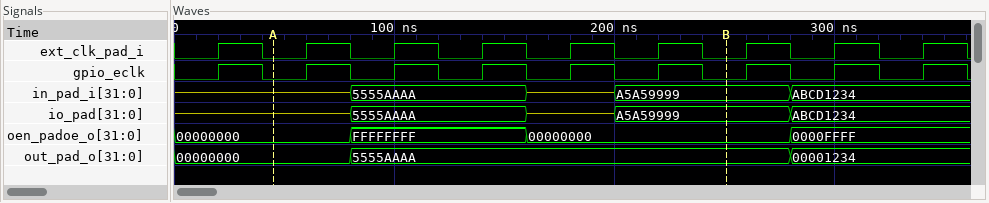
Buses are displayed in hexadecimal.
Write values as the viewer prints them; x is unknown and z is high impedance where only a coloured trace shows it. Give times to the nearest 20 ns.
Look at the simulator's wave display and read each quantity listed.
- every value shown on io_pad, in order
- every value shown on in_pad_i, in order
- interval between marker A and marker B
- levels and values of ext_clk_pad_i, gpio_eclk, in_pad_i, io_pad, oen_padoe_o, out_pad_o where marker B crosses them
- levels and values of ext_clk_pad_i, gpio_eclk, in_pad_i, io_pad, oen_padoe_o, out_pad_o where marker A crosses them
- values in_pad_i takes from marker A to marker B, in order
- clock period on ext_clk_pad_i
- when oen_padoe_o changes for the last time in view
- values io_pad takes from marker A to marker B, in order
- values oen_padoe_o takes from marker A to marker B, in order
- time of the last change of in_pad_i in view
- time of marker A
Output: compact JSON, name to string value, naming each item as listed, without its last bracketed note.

{"every value shown on io_pad, in order": "z, 5555AAAA, z, A5A59999, ABCD1234", "every value shown on in_pad_i, in order": "z, 5555AAAA, z, A5A59999, ABCD1234", "interval between marker A and marker B": "200 ns", "levels and values of ext_clk_pad_i, gpio_eclk, in_pad_i, io_pad, oen_padoe_o, out_pad_o where marker B crosses them": "ext_clk_pad_i=0, gpio_eclk=0, in_pad_i=A5A59999, io_pad=A5A59999, oen_padoe_o=00000000, out_pad_o=5555AAAA", "levels and values of ext_clk_pad_i, gpio_eclk, in_pad_i, io_pad, oen_padoe_o, out_pad_o where marker A crosses them": "ext_clk_pad_i=0, gpio_eclk=0, in_pad_i=z, io_pad=z, oen_padoe_o=00000000, out_pad_o=00000000", "values in_pad_i takes from marker A to marker B, in order": "z, 5555AAAA, z, A5A59999", "clock period on ext_clk_pad_i": "40 ns", "when oen_padoe_o changes for the last time in view": "280 ns", "values io_pad takes from marker A to marker B, in order": "z, 5555AAAA, z, A5A59999", "values oen_padoe_o takes from marker A to marker B, in order": "00000000, FFFFFFFF, 00000000", "time of the last change of in_pad_i in view": "280 ns", "time of marker A": "40 ns"}
